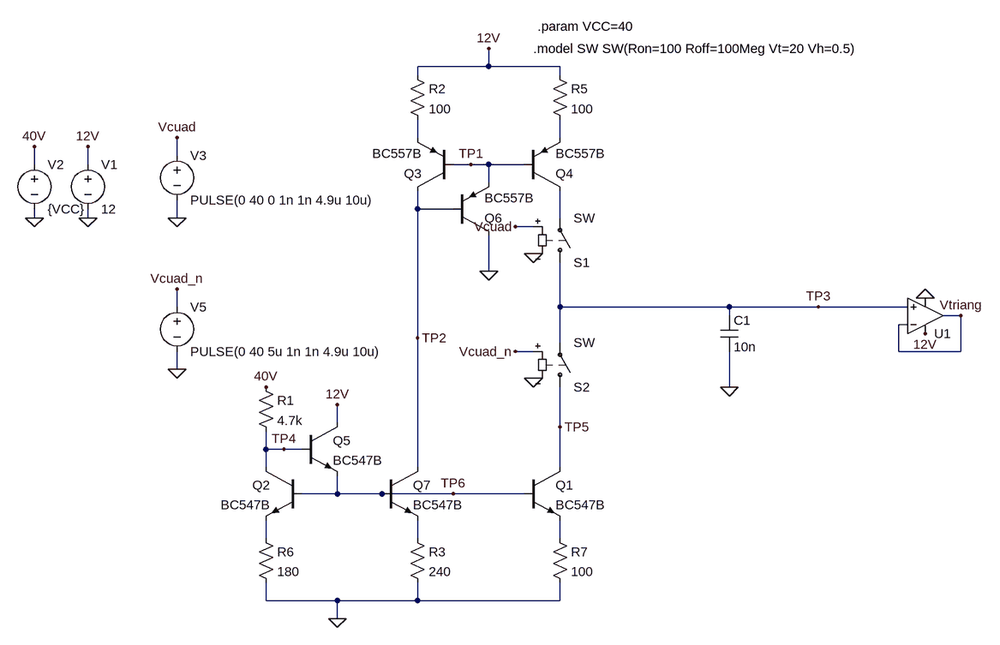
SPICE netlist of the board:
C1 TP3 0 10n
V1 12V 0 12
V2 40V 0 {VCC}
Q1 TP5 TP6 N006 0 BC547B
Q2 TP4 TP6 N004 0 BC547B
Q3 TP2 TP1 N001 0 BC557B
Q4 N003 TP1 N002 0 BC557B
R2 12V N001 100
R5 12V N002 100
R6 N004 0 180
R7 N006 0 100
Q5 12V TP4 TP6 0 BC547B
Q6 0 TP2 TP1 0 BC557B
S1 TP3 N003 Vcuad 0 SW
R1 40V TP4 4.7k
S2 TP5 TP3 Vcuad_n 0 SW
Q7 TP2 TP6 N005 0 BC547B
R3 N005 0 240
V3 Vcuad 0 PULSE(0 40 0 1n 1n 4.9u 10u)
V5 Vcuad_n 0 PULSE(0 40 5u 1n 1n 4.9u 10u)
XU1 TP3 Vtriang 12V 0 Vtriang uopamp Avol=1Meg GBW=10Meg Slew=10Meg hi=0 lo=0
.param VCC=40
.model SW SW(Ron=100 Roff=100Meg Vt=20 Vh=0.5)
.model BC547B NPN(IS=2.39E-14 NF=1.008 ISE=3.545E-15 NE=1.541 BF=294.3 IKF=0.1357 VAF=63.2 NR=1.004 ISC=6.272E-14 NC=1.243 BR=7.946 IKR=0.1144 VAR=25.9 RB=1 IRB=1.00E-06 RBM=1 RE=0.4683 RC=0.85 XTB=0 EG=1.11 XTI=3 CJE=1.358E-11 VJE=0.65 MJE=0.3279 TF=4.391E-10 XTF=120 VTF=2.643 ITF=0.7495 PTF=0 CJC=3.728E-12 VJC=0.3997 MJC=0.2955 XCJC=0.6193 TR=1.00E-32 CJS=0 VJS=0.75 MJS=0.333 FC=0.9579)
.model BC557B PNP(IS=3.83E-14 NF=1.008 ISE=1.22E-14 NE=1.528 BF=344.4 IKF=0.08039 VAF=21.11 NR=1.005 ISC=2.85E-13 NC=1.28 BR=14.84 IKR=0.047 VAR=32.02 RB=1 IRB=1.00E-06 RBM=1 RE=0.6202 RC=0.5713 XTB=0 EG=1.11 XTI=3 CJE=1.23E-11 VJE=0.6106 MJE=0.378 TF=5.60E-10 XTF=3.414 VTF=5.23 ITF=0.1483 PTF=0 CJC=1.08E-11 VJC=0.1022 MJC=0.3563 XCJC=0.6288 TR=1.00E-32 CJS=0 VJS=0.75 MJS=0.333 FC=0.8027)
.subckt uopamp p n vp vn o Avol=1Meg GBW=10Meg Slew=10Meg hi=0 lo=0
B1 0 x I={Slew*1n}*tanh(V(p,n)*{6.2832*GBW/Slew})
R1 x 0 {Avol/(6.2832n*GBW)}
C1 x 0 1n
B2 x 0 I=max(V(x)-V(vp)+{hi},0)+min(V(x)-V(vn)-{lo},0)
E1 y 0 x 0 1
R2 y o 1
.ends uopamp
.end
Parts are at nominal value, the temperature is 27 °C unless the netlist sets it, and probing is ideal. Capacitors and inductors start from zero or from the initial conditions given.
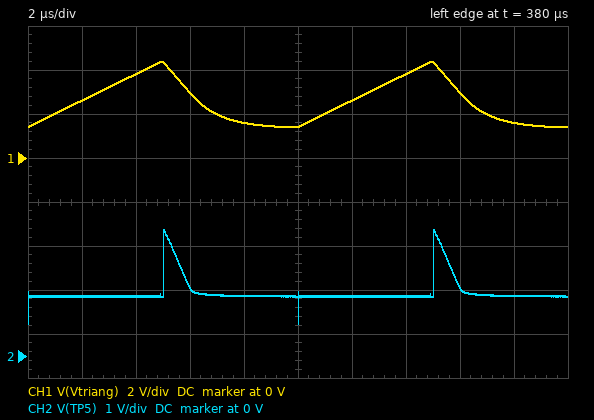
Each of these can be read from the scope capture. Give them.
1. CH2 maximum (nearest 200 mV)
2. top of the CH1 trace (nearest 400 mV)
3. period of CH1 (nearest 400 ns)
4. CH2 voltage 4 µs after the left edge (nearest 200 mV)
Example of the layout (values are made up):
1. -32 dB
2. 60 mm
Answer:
1. 2.8 V
2. 4.4 V
3. 10.0 µs
4. 1.4 V
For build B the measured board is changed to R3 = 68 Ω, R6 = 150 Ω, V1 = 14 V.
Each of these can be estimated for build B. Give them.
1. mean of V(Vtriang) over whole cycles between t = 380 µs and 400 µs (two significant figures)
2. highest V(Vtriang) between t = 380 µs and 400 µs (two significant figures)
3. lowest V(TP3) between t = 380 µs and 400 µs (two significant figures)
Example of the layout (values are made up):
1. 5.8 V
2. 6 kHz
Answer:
1. 9.6 V
2. 12 V
3. 6.3 V
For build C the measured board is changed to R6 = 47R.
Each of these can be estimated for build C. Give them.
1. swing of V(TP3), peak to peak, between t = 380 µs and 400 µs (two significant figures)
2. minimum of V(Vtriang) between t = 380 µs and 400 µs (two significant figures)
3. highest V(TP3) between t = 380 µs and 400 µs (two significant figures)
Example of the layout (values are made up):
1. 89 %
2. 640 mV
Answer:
1. 950 mV
2. 380 mV
3. 1.3 V
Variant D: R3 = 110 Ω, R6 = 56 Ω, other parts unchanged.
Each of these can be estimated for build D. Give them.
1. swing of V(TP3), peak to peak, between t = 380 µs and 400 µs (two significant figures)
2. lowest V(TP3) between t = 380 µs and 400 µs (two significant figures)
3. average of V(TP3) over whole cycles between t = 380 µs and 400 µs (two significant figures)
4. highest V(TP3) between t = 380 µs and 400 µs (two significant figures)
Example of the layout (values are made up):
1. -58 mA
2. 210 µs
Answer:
1. 2.2 V
2. 670 mV
3. 1.7 V
4. 2.9 V
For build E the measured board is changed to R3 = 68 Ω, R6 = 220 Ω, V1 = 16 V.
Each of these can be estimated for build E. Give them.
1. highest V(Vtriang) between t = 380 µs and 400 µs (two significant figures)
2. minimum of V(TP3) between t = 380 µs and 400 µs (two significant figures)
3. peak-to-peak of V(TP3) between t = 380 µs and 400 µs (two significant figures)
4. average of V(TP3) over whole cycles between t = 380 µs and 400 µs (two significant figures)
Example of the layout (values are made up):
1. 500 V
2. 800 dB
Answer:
1. 13 V
2. 4.9 V
3. 8.4 V
4. 9.7 V
